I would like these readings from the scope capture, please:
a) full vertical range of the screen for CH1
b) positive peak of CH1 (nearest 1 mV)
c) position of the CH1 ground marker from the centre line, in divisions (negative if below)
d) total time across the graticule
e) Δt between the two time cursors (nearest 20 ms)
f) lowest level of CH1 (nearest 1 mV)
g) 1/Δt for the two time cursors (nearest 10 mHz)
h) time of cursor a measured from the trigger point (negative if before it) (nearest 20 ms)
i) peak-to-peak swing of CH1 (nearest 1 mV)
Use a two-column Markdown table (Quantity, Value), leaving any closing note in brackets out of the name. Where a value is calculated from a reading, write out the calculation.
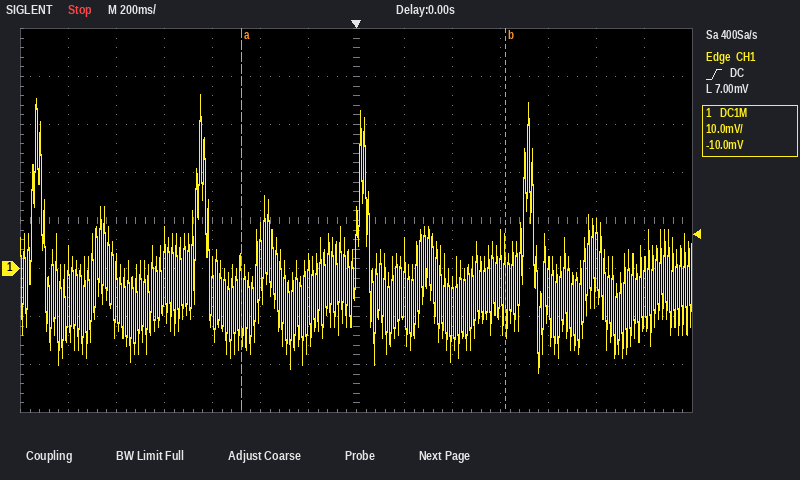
| Quantity | Value |
|---|---|
| full vertical range of the screen for CH1 | 80 mV |
| positive peak of CH1 | 36 mV |
| position of the CH1 ground marker from the centre line, in divisions | -1.0 div |
| total time across the graticule | 2.8 s |
| Δt between the two time cursors | 1.10 s |
| lowest level of CH1 | -22 mV |
| 1/Δt for the two time cursors | 1 / 1.10 s ≈ 910 mHz |
| time of cursor a measured from the trigger point (negative if before it) | -480 ms |
| peak-to-peak swing of CH1 | 36 mV − (-22 mV) = 58 mV |
